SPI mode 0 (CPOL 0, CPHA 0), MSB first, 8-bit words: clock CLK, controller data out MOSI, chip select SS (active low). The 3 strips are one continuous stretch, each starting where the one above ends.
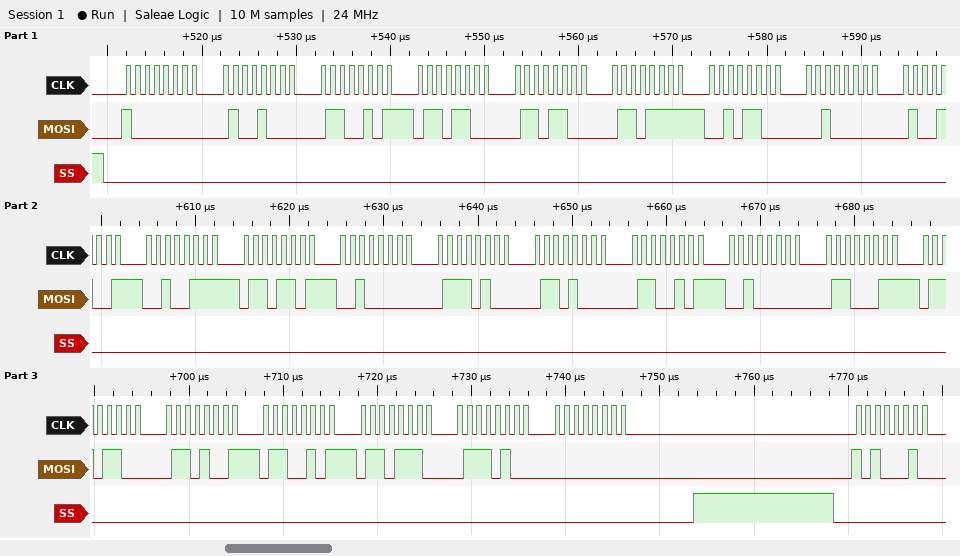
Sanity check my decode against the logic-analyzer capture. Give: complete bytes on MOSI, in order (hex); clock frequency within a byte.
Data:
80 48 65 6C 6C 6F 2C 20 49 27 6D 20 74 68 65 20 63 6C 69 65 6E 74 00 A2
1 MHz
